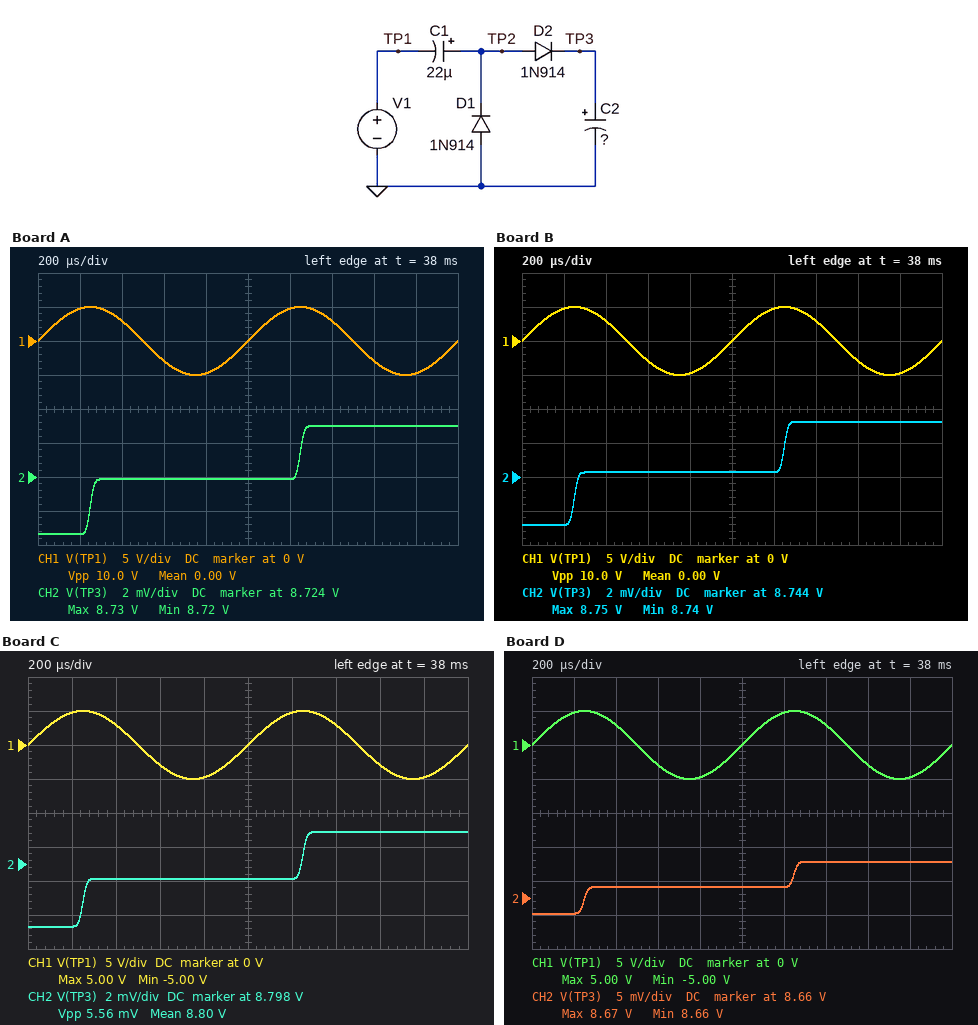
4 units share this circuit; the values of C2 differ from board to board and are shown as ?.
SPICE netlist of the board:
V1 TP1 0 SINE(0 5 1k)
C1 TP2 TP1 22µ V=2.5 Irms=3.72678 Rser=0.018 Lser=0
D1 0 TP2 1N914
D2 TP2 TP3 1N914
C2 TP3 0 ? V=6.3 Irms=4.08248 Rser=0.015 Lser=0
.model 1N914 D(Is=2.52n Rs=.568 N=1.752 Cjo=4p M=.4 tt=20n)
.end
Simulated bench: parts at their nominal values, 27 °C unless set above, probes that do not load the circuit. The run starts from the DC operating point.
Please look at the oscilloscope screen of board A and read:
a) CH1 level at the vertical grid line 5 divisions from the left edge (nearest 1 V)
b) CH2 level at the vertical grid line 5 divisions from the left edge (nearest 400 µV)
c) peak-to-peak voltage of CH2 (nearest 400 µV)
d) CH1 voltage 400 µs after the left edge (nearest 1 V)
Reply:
0 V
8.7240 V
6.4 mV
3 V
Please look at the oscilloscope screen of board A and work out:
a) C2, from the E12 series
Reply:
33 µF
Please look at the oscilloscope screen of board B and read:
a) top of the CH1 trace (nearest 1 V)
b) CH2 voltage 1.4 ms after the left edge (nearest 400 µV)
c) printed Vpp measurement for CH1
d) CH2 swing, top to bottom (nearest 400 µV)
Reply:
5 V
8.7472 V
10.0 V
6.0 mV
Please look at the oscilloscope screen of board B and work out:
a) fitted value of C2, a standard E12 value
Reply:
27 µF
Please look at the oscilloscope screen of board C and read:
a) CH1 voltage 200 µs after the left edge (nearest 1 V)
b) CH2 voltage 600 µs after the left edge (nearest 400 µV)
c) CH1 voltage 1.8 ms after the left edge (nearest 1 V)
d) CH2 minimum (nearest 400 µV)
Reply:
5 V
8.7972 V
-5 V
8.7944 V
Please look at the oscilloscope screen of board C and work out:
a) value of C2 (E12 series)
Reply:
15 µF
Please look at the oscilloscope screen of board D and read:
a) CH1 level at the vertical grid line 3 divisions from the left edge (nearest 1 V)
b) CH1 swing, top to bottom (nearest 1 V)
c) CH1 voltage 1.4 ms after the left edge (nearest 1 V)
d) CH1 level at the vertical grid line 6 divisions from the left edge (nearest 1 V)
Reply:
-3 V
10 V
3 V
5 V
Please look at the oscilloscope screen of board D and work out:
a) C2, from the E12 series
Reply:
56 µF
